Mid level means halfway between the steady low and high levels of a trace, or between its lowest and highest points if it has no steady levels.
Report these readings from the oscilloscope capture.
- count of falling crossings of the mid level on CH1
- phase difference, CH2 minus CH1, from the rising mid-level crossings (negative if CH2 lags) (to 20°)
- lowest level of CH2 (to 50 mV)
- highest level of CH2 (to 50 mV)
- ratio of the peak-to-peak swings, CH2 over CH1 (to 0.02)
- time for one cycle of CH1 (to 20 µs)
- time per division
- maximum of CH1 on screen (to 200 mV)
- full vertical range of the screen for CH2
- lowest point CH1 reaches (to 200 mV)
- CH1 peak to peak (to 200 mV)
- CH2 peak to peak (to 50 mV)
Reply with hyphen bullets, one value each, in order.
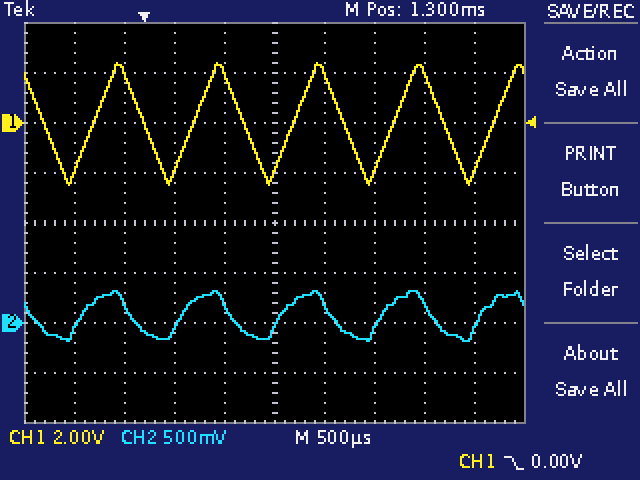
- 5
- +40°
- -200 mV
- 300 mV
- 0.10
- 1.00 ms
- 500 µs
- 2.4 V
- 4 V
- -2.4 V
- 4.8 V
- 500 mV
